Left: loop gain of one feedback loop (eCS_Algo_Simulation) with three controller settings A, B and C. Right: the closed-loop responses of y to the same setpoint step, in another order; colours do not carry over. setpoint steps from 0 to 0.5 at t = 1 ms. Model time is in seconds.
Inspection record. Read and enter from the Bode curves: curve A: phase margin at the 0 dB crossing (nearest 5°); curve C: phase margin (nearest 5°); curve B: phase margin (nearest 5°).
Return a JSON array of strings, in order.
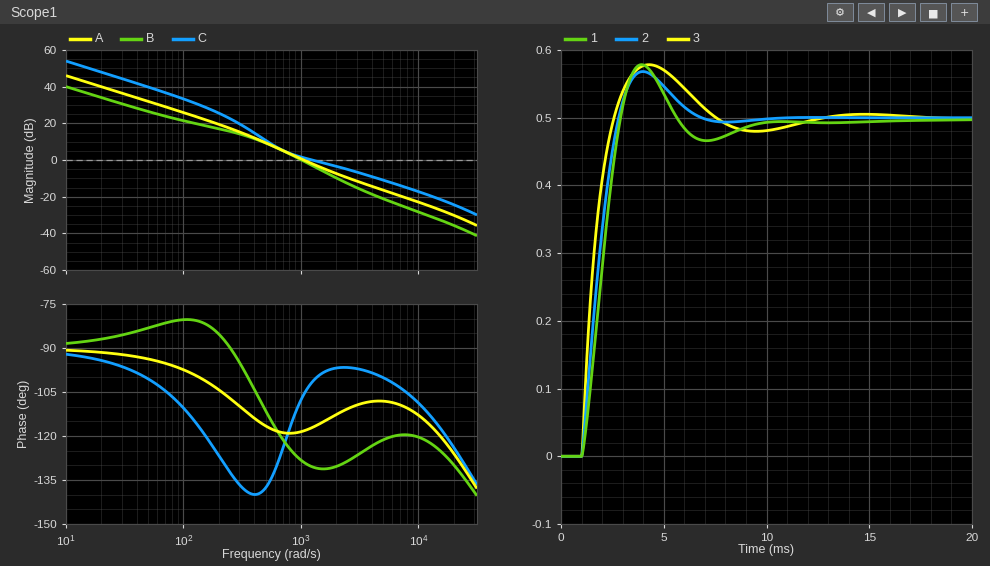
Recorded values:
["60°", "80°", "50°"]
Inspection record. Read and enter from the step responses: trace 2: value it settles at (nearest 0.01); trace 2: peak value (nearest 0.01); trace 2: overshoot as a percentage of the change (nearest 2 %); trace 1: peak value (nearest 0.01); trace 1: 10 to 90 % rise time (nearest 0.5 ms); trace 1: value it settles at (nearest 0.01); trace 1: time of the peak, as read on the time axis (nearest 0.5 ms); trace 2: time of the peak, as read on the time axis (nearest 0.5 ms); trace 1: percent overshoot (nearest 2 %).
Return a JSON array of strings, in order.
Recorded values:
["0.50", "0.57", "14 %", "0.58", "1.5 ms", "0.50", "4.0 ms", "4.0 ms", "16 %"]
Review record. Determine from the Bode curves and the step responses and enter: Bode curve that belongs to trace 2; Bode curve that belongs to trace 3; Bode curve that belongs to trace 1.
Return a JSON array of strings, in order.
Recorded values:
["A", "C", "B"]
